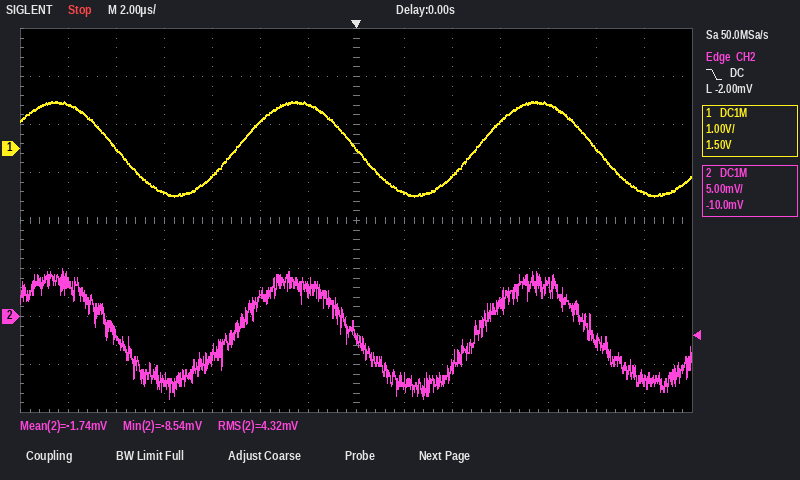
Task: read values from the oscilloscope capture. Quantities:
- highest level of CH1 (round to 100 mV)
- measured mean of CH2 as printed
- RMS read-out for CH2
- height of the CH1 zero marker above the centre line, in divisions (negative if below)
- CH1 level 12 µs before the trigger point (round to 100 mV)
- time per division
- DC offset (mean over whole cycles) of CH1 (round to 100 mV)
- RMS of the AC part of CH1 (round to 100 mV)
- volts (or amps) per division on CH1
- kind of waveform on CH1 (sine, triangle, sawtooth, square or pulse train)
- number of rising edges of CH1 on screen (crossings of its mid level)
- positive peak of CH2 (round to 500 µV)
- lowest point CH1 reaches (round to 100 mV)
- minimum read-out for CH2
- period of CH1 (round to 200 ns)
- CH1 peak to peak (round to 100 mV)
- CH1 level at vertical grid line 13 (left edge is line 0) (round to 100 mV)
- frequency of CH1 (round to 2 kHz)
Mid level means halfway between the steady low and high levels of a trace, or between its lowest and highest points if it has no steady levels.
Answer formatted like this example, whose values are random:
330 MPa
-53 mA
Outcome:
1.0 V
-1.74 mV
4.32 mV
+1.5 div
900 mV
2 µs
0.0 V
700 mV
1 V
sine
2
5.0 mV
-1.0 V
-8.54 mV
10.0 µs
2.0 V
-900 mV
100 kHz
